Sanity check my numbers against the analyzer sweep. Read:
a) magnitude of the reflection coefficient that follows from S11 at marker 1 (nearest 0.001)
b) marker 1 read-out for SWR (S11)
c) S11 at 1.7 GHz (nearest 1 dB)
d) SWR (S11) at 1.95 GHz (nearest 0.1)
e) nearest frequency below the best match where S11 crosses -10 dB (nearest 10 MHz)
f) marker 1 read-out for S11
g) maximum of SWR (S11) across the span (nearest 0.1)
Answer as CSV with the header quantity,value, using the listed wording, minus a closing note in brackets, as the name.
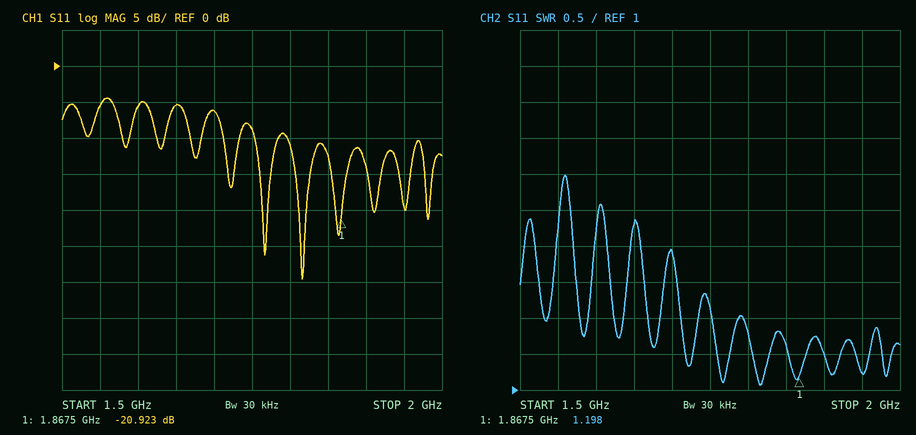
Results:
quantity,value
magnitude of the reflection coefficient that follows from S11 at marker 1,0.090
marker 1 read-out for SWR,1.198
S11 at 1.7 GHz,-6 dB
SWR (S11) at 1.95 GHz,1.2
nearest frequency below the best match where S11 crosses -10 dB,1.80 GHz
marker 1 read-out for S11,-20.923 dB
maximum of SWR (S11) across the span,4.0
